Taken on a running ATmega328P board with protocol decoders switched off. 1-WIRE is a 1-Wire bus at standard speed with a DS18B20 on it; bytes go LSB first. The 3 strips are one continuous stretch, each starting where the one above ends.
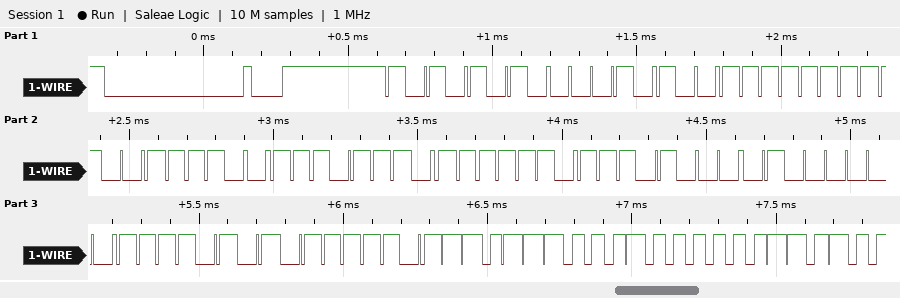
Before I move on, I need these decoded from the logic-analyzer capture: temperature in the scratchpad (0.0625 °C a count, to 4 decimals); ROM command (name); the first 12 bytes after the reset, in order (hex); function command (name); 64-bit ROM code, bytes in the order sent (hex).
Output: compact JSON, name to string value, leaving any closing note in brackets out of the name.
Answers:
{"temperature in the scratchpad": "35.6875 °C", "ROM command": "Match ROM", "the first 12 bytes after the reset, in order": "55 28 FF 79 EE 7E 17 02 AF BE 3B 02", "function command": "Read Scratchpad", "64-bit ROM code, bytes in the order sent": "28 FF 79 EE 7E 17 02 AF"}
